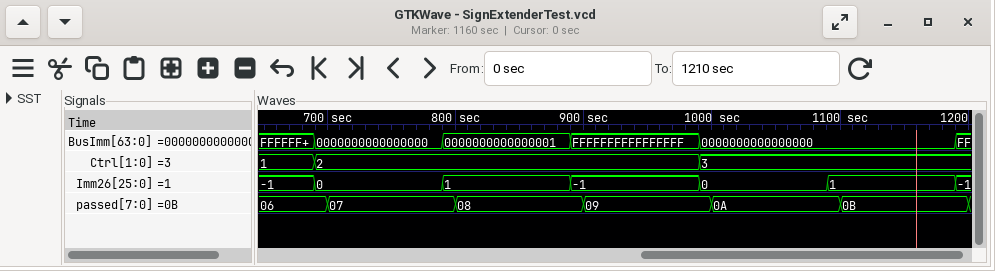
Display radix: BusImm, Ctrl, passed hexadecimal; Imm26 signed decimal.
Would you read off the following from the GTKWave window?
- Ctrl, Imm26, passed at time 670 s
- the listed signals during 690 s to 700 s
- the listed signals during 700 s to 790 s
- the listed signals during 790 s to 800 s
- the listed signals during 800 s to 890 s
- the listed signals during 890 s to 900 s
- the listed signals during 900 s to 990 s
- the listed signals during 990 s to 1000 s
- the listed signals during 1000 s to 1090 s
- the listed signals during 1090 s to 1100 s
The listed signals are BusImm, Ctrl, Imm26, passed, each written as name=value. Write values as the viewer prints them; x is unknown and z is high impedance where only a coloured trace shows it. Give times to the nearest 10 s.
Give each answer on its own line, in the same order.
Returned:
Ctrl=1, Imm26=-1, passed=06
BusImm=0000000000000000, Ctrl=2, Imm26=0, passed=06
BusImm=0000000000000000, Ctrl=2, Imm26=0, passed=07
BusImm=0000000000000001, Ctrl=2, Imm26=1, passed=07
BusImm=0000000000000001, Ctrl=2, Imm26=1, passed=08
BusImm=FFFFFFFFFFFFFFFF, Ctrl=2, Imm26=-1, passed=08
BusImm=FFFFFFFFFFFFFFFF, Ctrl=2, Imm26=-1, passed=09
BusImm=0000000000000000, Ctrl=3, Imm26=0, passed=09
BusImm=0000000000000000, Ctrl=3, Imm26=0, passed=0A
BusImm=0000000000000000, Ctrl=3, Imm26=1, passed=0A
